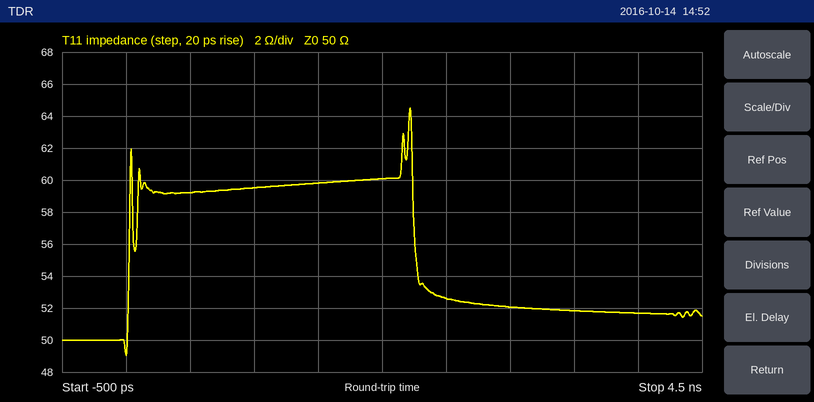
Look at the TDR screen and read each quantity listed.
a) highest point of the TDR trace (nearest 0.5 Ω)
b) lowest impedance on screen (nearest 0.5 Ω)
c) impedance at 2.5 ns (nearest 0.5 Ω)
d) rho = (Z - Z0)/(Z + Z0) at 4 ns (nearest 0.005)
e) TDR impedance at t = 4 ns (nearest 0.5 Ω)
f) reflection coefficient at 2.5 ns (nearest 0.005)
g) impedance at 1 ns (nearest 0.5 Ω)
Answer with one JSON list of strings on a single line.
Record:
["64.5 Ω", "49.0 Ω", "52.5 Ω", "+0.015", "51.5 Ω", "+0.025", "59.5 Ω"]
